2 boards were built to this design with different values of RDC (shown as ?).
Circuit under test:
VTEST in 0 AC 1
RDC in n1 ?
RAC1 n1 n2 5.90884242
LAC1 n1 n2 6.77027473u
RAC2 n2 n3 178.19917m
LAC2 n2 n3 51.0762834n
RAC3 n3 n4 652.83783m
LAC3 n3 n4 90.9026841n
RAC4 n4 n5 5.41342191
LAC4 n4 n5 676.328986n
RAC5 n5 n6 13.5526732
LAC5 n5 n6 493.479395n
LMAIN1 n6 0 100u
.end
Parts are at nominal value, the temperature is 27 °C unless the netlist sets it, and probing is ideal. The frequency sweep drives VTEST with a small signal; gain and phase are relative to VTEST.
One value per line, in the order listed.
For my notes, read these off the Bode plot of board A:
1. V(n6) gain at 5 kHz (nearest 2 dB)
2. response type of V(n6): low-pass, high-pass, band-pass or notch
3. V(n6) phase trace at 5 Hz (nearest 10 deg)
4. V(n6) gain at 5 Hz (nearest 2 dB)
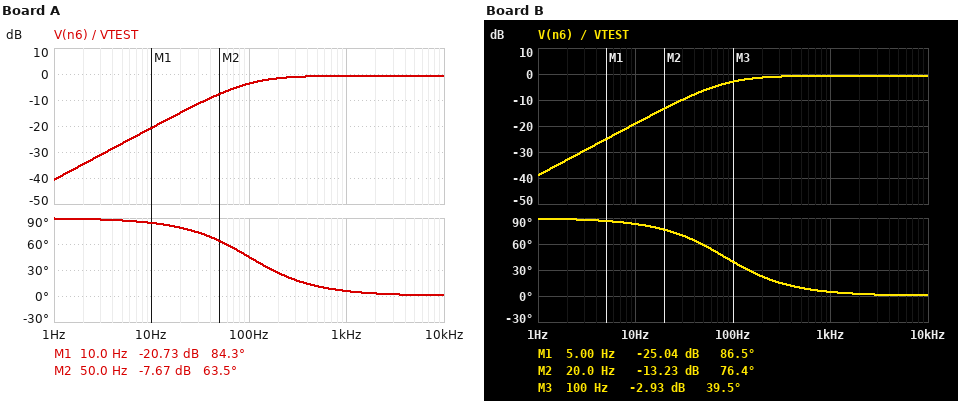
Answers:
0 dB
high-pass
90 deg
-26 dB
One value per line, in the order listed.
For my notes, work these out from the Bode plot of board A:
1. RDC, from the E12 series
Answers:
0.068 Ω
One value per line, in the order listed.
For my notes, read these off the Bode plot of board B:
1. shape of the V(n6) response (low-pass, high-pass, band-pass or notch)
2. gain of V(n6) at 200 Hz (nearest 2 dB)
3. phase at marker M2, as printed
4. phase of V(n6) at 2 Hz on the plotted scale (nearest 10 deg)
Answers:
high-pass
-2 dB
76.4 deg
90 deg
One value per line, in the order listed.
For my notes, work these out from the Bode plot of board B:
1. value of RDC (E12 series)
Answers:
0.056 Ω
